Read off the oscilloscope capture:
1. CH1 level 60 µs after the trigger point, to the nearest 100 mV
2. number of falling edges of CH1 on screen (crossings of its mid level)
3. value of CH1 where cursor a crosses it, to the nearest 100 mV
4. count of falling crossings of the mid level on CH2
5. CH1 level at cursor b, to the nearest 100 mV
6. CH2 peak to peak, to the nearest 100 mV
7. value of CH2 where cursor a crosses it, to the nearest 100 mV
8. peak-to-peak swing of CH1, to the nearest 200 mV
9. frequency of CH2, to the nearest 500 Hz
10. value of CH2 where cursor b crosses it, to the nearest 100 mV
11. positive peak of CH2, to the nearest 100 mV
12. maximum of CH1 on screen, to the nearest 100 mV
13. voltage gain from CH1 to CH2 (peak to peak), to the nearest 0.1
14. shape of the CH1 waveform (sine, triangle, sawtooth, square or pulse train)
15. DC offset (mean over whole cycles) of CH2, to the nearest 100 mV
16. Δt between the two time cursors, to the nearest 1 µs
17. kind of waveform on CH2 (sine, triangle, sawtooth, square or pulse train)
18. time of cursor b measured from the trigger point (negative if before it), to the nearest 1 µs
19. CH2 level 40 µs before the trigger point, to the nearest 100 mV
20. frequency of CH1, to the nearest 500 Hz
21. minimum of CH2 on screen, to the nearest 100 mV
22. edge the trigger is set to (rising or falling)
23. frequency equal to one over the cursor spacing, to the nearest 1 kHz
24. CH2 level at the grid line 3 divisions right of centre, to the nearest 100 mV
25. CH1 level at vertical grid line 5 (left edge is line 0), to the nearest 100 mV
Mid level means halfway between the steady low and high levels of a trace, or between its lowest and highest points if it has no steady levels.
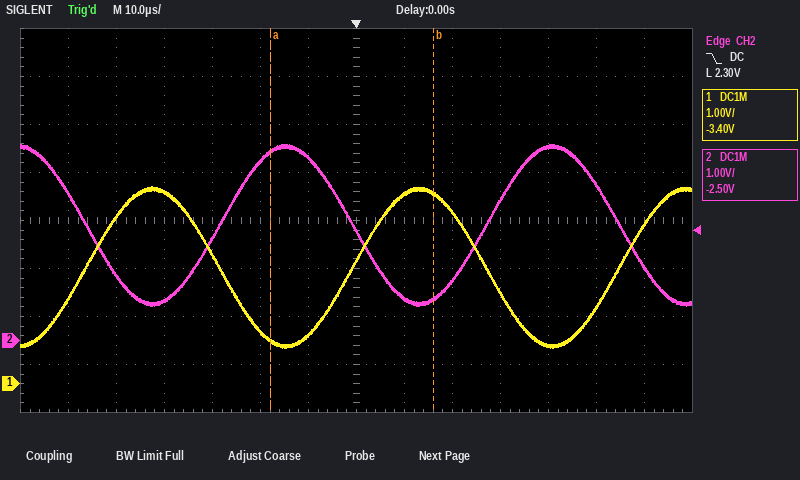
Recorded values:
3.3 V
2
900 mV
3
4.0 V
3.4 V
3.9 V
3.4 V
18.0 kHz
900 mV
4.1 V
4.1 V
1.0
sine
2.4 V
34 µs
sine
+16 µs
800 mV
18.0 kHz
700 mV
falling
29 kHz
2.9 V
1.1 V
